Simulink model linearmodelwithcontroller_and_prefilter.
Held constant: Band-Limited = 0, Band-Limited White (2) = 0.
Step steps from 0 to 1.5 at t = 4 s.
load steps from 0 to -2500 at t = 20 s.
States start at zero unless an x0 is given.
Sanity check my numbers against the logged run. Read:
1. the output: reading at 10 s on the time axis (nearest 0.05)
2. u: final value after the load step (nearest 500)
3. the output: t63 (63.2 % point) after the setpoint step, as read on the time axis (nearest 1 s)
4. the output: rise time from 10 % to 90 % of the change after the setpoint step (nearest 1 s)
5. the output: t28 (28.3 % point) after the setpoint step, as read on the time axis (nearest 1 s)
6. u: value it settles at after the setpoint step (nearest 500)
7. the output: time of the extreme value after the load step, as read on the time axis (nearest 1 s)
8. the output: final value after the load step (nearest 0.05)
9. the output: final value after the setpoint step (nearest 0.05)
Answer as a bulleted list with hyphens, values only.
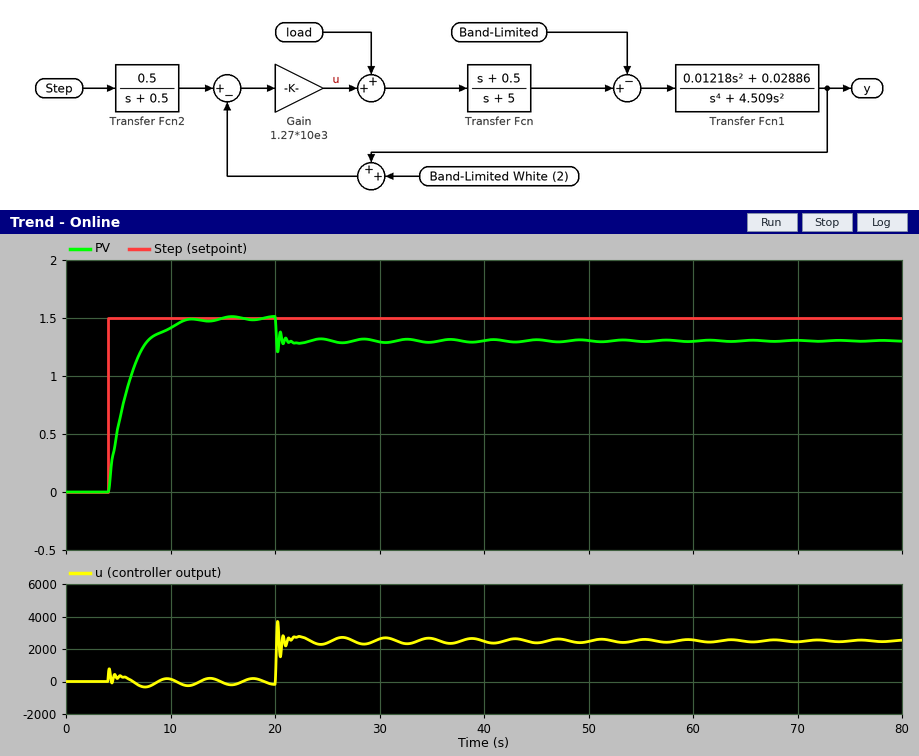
- 1.40
- 2500
- 6 s
- 4 s
- 5 s
- 0
- 20 s
- 1.30
- 1.50
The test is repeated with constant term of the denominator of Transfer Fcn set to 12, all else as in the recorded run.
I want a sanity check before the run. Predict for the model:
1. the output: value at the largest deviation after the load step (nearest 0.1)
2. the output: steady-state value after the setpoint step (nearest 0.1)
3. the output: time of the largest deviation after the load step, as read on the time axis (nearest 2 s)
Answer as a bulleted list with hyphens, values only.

- 1.3
- 1.5
- 22 s
